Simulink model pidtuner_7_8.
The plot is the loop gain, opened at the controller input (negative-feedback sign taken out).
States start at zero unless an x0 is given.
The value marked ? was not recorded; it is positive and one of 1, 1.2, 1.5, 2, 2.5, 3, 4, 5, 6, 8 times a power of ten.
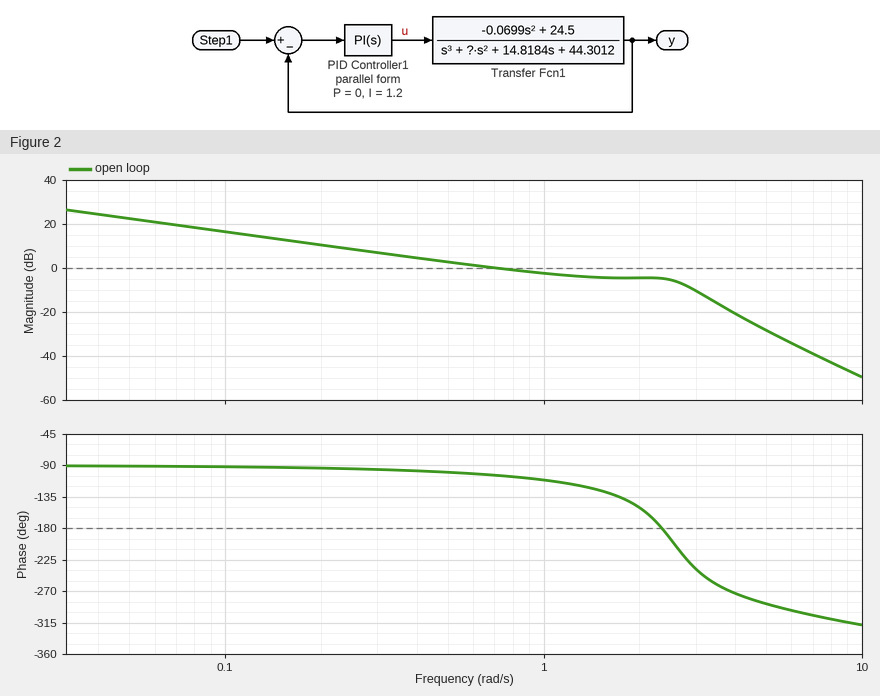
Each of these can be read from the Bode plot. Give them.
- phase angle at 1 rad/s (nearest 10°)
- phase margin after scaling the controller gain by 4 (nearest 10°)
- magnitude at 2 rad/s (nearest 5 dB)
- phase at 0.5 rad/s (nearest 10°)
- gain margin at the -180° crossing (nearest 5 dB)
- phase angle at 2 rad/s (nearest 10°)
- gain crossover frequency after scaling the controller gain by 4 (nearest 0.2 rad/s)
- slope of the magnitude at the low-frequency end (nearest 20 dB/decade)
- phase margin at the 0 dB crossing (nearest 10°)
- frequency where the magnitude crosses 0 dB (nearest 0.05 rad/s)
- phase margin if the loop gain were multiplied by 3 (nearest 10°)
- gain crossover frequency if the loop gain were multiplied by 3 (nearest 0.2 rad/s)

-110°
-70°
-5 dB
-100°
5 dB
-150°
3.2 rad/s
-20 dB/decade
80°
0.70 rad/s
-50°
3.0 rad/s
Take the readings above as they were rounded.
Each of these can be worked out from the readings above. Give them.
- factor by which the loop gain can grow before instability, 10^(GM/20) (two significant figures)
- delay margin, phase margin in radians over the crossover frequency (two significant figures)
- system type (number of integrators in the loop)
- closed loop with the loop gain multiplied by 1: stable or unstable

1.8
2.0 s
1
stable
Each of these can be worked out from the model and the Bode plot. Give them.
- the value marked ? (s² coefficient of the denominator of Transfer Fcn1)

8
